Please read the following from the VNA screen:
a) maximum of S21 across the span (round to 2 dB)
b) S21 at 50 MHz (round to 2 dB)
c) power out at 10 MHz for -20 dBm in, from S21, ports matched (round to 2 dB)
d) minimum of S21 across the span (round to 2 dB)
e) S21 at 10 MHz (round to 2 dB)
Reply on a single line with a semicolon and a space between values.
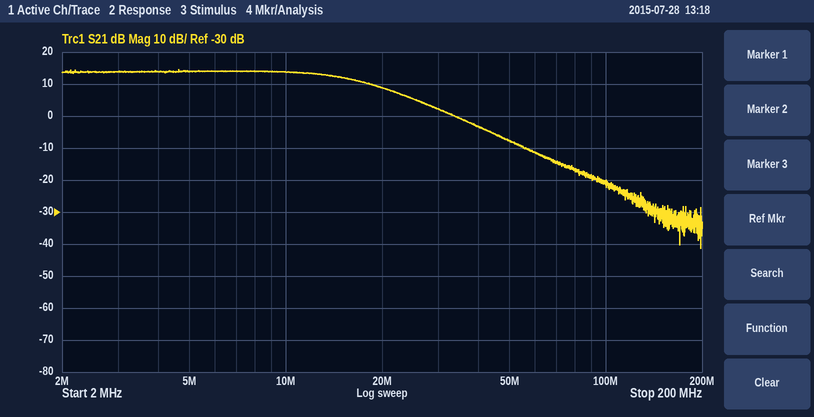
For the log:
14 dB; -8 dB; -6 dBm; -42 dB; 14 dB
